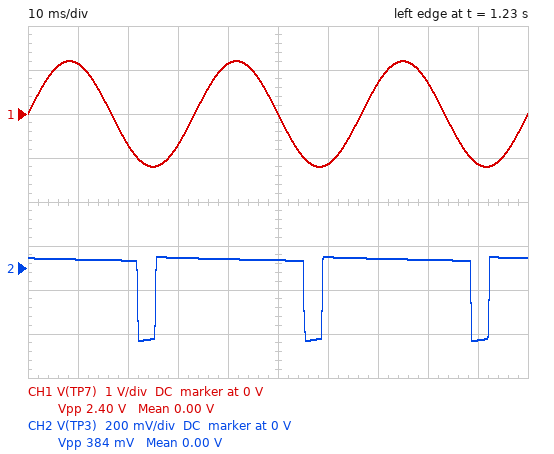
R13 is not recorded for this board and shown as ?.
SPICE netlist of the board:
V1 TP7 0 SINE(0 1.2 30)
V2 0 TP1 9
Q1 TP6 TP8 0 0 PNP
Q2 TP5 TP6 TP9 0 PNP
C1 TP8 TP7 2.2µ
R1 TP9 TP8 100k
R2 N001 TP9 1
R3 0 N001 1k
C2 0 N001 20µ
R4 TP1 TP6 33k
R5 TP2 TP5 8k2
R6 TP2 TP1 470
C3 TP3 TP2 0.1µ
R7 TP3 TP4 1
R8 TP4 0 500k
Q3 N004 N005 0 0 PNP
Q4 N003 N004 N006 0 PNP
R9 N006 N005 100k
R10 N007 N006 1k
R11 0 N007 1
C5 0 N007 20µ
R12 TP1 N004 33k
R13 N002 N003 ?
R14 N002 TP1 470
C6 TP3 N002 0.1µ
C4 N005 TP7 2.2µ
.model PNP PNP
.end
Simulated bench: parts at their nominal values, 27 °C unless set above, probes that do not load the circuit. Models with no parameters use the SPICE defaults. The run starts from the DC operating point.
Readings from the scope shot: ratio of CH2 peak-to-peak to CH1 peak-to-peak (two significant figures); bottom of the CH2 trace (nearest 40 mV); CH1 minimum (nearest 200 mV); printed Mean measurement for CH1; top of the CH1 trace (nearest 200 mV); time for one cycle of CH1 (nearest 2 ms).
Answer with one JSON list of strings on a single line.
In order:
["0.16", "-320 mV", "-1.2 V", "0.00 V", "1.2 V", "34 ms"]
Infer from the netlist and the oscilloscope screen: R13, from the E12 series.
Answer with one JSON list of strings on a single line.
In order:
["12 kΩ"]
